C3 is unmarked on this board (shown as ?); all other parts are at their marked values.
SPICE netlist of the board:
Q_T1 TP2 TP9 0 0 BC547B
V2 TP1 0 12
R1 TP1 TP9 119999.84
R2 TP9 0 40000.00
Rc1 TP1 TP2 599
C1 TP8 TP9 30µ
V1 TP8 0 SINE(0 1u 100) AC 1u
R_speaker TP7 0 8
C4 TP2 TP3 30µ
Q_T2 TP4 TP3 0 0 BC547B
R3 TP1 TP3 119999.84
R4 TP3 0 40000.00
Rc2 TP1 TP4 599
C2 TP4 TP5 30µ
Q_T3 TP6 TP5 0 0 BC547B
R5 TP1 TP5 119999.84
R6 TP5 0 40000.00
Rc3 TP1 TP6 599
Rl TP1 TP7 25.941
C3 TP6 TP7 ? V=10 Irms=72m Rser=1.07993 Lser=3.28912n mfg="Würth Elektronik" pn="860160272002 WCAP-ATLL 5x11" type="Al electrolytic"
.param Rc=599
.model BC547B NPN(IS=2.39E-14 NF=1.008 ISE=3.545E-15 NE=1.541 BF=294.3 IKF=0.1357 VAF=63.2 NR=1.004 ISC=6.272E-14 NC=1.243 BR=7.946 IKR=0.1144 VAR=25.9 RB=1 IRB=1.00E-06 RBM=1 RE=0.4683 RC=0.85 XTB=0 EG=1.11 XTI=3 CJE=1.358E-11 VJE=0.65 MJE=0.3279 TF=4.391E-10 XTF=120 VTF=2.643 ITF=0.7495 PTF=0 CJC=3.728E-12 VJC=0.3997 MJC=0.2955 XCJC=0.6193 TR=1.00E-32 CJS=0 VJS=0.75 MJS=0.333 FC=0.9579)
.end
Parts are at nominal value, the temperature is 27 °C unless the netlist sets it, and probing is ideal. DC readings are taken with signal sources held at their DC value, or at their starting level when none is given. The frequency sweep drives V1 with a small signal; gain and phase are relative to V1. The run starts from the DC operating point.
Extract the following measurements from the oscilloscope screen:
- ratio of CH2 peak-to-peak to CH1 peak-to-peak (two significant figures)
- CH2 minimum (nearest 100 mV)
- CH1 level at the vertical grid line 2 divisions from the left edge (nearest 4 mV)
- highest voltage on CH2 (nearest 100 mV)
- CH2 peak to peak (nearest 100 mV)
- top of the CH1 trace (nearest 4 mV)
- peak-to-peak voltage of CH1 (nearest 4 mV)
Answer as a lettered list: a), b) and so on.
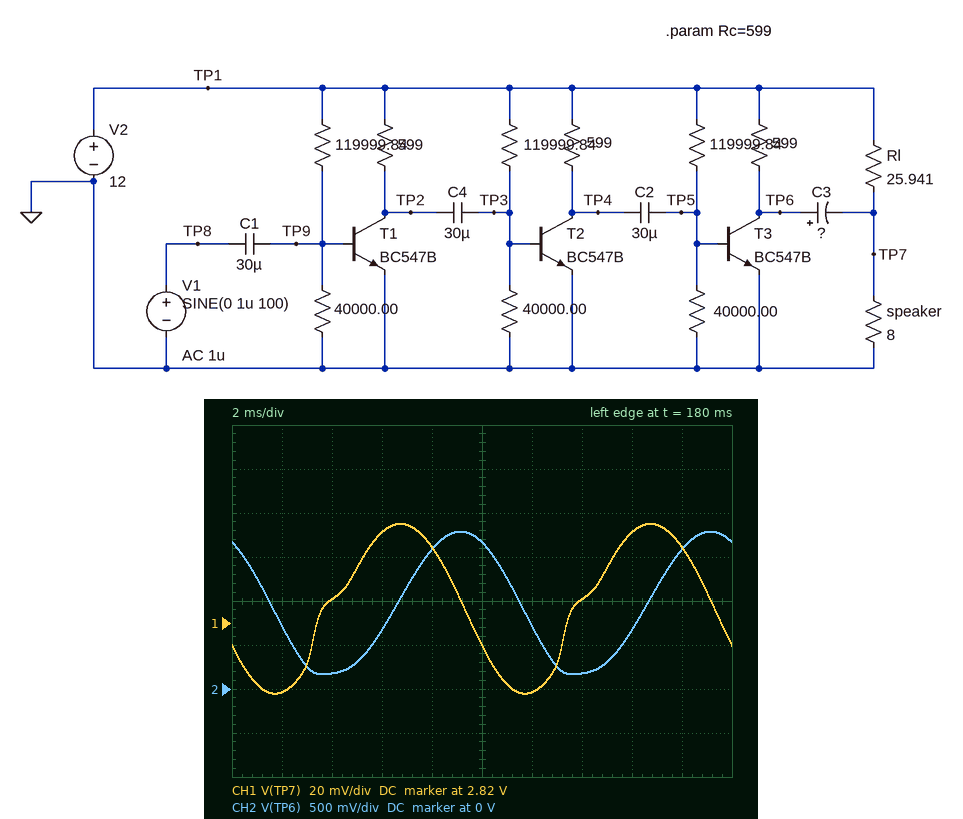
a) 21
b) 200 mV
c) 2.832 V
d) 1.8 V
e) 1.6 V
f) 2.864 V
g) 76 mV
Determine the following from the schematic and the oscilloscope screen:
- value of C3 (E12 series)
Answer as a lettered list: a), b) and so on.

a) 12 µF
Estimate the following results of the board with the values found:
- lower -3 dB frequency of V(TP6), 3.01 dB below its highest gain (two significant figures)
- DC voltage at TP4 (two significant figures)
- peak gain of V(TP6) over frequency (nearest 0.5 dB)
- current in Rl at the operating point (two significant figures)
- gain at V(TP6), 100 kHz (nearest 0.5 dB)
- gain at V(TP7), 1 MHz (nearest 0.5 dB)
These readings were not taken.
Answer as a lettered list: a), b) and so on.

a) 9.8 Hz
b) 690 mV
c) 127.0 dB
d) 350 mA
e) 93.5 dB
f) 86.5 dB
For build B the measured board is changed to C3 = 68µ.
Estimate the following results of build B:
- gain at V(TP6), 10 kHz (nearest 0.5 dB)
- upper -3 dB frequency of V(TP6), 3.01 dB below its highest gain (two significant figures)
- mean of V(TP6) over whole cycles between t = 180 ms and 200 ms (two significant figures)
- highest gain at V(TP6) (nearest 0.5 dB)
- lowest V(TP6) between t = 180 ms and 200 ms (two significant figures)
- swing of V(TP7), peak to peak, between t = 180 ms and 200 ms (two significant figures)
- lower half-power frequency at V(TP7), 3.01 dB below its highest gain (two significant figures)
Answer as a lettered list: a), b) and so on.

a) 93.5 dB
b) 27 Hz
c) 750 mV
d) 117.0 dB
e) 590 mV
f) 80 mV
g) 17 Hz
